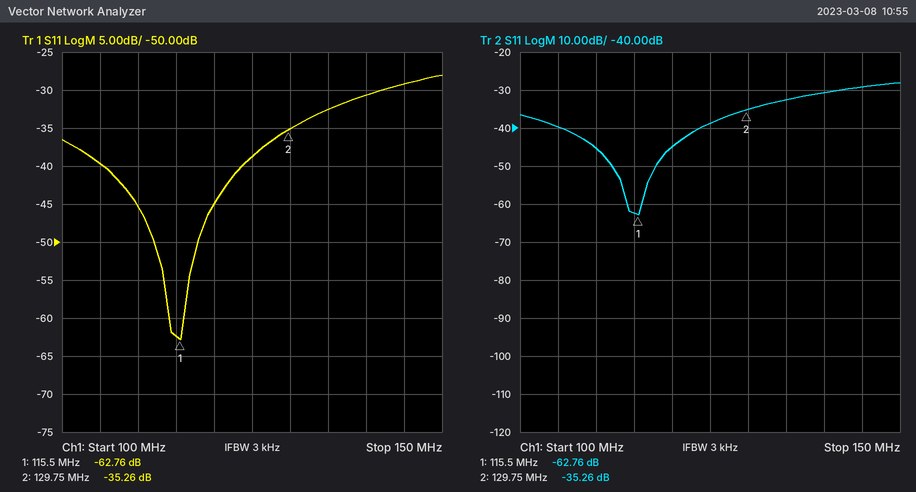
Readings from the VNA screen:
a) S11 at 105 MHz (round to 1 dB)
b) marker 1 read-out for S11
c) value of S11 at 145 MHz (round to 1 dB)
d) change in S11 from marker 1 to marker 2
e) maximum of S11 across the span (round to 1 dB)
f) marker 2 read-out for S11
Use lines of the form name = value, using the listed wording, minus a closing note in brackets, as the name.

S11 at 105 MHz = -40 dB
marker 1 read-out for S11 = -62.76 dB
value of S11 at 145 MHz = -29 dB
change in S11 from marker 1 to marker 2 = 27.50 dB
maximum of S11 across the span = -28 dB
marker 2 read-out for S11 = -35.26 dB
